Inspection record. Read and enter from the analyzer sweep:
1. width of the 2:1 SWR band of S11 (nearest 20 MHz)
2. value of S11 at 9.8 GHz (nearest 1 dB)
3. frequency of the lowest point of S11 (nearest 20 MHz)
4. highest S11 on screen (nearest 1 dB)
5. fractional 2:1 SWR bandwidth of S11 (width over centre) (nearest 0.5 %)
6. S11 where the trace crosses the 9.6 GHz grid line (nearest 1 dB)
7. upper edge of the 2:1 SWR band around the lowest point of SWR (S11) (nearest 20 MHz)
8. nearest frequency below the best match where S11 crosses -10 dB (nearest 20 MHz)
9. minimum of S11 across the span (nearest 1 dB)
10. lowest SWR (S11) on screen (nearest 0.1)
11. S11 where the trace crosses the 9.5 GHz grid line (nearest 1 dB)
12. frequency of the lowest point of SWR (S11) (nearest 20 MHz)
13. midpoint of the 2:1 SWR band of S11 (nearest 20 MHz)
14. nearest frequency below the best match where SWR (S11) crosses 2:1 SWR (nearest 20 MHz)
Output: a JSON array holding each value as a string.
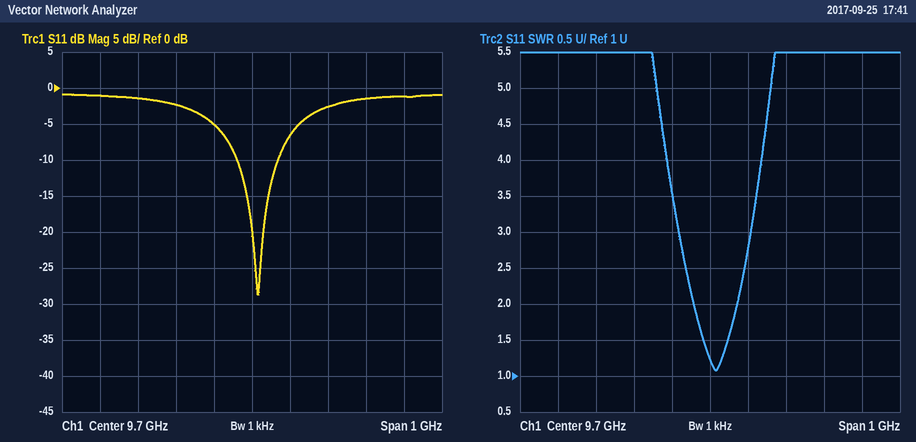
["120 MHz", "-7 dB", "9.72 GHz", "-1 dB", "1.0 %", "-5 dB", "9.78 GHz", "9.66 GHz", "-29 dB", "1.1", "-2 dB", "9.72 GHz", "9.72 GHz", "9.66 GHz"]
